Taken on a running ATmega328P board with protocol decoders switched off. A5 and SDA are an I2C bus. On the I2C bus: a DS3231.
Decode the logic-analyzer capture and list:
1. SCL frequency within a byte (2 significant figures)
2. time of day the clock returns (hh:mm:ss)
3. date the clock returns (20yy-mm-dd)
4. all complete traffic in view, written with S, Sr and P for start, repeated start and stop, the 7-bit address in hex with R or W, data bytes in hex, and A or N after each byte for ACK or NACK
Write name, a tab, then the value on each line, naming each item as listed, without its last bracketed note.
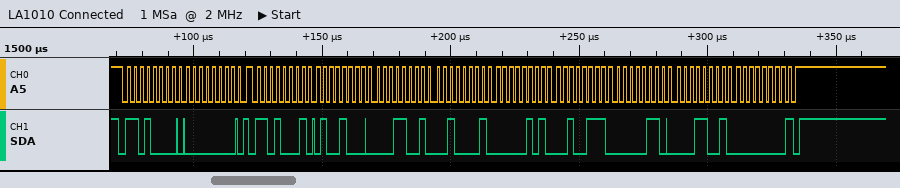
SCL frequency within a byte	400 kHz
time of day the clock returns	21:19:48
date the clock returns	2019-06-27
all complete traffic in view, written with S, Sr and P for start, repeated start and stop, the 7-bit address in hex with R or W, data bytes in hex, and A or N after each byte for ACK or NACK	S 68W A 00 A Sr 68R A 48 A 19 A 21 A 05 A 27 A 06 A 19 A 00 N P
